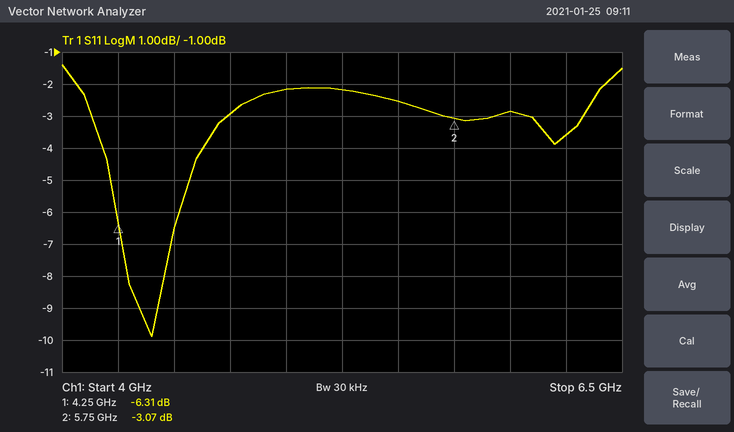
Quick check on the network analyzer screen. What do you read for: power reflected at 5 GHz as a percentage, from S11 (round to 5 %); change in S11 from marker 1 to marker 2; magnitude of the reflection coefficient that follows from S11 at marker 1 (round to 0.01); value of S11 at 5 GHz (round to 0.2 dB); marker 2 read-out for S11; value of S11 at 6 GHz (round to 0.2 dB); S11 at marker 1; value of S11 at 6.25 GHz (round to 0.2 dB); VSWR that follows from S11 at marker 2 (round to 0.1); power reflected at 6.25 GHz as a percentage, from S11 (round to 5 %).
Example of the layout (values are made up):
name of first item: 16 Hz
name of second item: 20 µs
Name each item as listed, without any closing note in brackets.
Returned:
power reflected at 5 GHz as a percentage, from S11: 60 %
change in S11 from marker 1 to marker 2: 3.24 dB
magnitude of the reflection coefficient that follows from S11 at marker 1: 0.48
value of S11 at 5 GHz: -2.2 dB
marker 2 read-out for S11: -3.07 dB
value of S11 at 6 GHz: -2.8 dB
S11 at marker 1: -6.31 dB
value of S11 at 6.25 GHz: -3.6 dB
VSWR that follows from S11 at marker 2: 5.7
power reflected at 6.25 GHz as a percentage, from S11: 45 %
